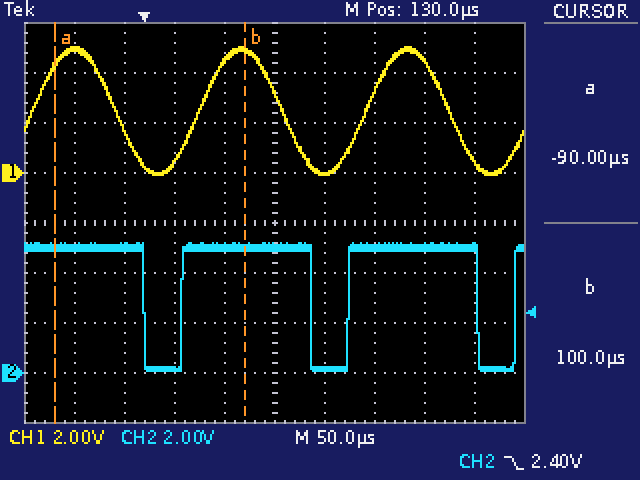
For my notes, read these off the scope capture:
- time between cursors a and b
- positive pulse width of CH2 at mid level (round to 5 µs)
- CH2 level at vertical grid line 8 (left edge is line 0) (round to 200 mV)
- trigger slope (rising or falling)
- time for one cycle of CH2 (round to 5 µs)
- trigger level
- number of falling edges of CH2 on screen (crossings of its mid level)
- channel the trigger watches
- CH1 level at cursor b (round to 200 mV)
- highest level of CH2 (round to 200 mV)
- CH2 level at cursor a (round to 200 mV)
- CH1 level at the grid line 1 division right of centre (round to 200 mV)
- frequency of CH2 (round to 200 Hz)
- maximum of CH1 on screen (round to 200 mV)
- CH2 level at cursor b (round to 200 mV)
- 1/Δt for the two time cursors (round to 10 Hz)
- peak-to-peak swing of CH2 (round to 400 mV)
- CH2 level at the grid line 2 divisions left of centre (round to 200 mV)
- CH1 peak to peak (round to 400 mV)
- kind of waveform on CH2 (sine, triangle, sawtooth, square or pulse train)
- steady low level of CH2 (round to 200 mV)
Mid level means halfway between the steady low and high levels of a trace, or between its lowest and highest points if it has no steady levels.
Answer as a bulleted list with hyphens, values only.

- 190 µs
- 130 µs
- 5.0 V
- falling
- 165 µs
- 2.40 V
- 3
- CH2
- 4.8 V
- 5.2 V
- 5.0 V
- 0.0 V
- 6.0 kHz
- 5.0 V
- 5.0 V
- 5.26 kHz
- 5.2 V
- 200 mV
- 5.2 V
- pulse train
- 200 mV
